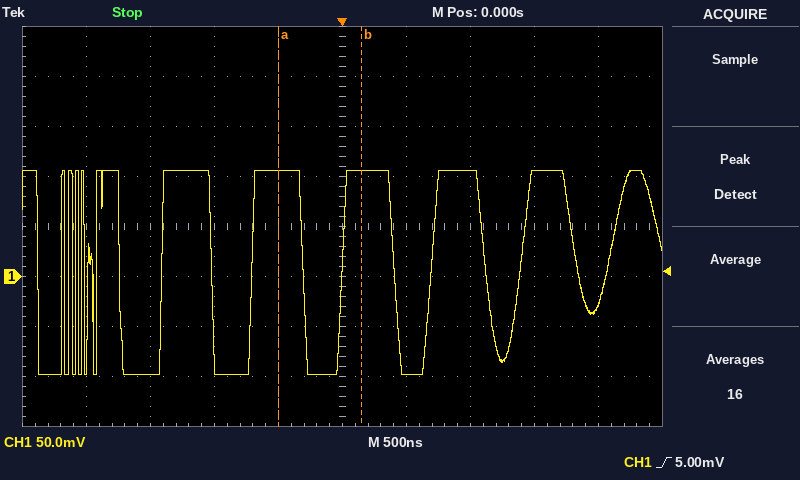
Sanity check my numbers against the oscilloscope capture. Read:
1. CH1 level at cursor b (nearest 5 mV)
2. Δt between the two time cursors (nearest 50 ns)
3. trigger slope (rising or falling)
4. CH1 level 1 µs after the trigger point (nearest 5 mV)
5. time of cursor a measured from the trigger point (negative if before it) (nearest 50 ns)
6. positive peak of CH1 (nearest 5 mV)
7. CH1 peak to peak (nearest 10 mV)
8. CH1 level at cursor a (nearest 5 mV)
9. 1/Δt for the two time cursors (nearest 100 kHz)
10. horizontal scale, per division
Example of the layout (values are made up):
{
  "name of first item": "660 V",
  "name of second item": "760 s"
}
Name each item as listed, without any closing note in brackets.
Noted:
{
  "CH1 level at cursor b": "105 mV",
  "Δt between the two time cursors": "650 ns",
  "trigger slope": "rising",
  "CH1 level 1 µs after the trigger point": "105 mV",
  "time of cursor a measured from the trigger point (negative if before it)": "-500 ns",
  "positive peak of CH1": "105 mV",
  "CH1 peak to peak": "200 mV",
  "CH1 level at cursor a": "105 mV",
  "1/Δt for the two time cursors": "1.5 MHz",
  "horizontal scale, per division": "500 ns"
}
